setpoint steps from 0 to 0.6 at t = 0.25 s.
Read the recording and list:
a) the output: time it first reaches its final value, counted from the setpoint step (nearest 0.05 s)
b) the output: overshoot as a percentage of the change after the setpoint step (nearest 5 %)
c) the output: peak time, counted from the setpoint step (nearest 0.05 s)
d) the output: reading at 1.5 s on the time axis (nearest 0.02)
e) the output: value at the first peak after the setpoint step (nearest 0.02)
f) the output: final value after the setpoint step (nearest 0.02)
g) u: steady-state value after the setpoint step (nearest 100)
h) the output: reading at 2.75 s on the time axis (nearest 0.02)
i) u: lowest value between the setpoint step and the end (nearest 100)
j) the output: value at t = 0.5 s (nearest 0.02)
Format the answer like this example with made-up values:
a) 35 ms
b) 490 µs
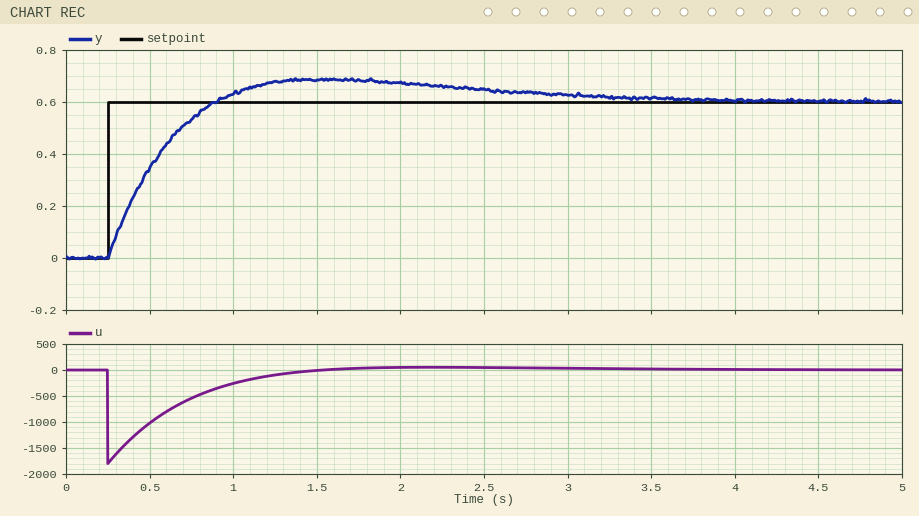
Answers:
a) 0.65 s
b) 15 %
c) 1.30 s
d) 0.68
e) 0.68
f) 0.60
g) 0
h) 0.64
i) -1800
j) 0.34
